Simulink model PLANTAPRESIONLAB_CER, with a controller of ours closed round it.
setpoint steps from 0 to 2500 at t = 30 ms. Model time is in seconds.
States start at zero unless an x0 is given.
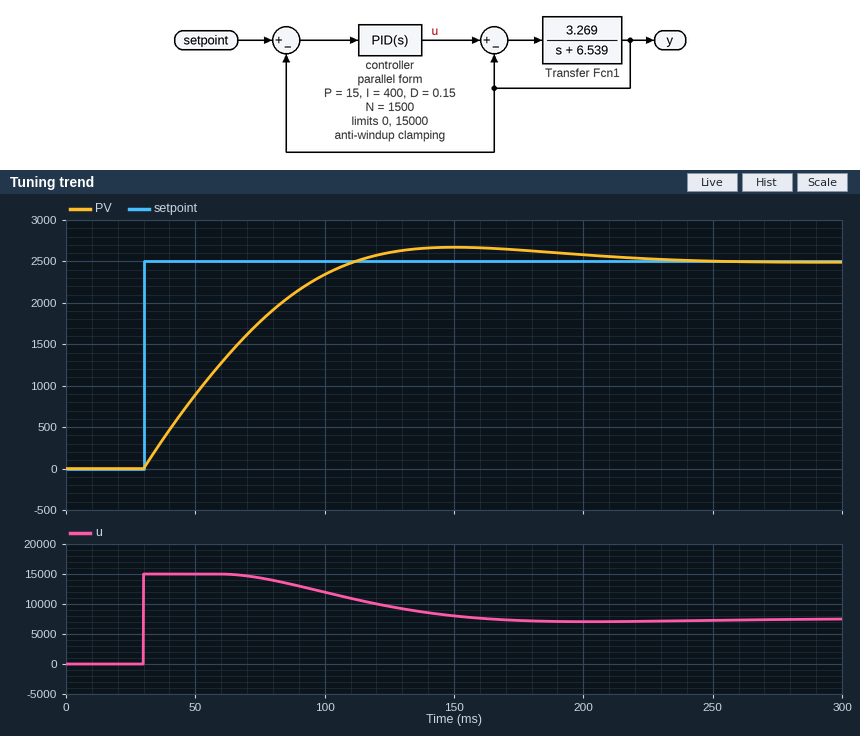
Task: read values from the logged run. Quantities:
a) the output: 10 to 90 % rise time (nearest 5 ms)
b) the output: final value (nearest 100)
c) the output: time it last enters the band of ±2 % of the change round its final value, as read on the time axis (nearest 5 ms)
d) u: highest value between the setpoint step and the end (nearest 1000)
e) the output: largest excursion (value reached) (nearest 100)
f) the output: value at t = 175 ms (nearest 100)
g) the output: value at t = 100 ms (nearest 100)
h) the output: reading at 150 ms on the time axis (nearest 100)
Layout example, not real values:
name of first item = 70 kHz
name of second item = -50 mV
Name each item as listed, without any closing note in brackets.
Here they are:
the output: 10 to 90 % rise time = 60 ms
the output: final value = 2500
the output: time it last enters the band of ±2 % of the change round its final value, as read on the time axis = 215 ms
u: highest value between the setpoint step and the end = 15000
the output: largest excursion (value reached) = 2700
the output: value at t = 175 ms = 2600
the output: value at t = 100 ms = 2300
the output: reading at 150 ms on the time axis = 2700
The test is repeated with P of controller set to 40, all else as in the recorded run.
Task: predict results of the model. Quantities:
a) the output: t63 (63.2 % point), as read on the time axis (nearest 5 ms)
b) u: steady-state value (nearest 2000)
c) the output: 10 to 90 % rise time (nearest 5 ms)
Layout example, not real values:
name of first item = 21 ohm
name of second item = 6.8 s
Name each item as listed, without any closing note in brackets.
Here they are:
the output: t63 (63.2 % point), as read on the time axis = 70 ms
u: steady-state value = 8000
the output: 10 to 90 % rise time = 60 ms
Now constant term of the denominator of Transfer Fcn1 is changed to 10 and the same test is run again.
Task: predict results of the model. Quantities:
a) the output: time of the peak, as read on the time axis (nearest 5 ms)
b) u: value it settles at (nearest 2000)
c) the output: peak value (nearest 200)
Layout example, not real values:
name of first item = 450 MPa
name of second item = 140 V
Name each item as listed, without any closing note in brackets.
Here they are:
the output: time of the peak, as read on the time axis = 165 ms
u: value it settles at = 10000
the output: peak value = 2600
